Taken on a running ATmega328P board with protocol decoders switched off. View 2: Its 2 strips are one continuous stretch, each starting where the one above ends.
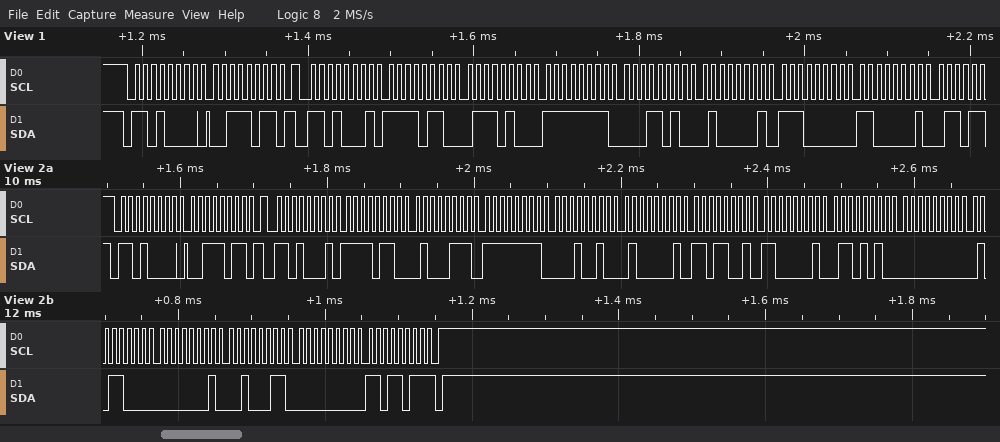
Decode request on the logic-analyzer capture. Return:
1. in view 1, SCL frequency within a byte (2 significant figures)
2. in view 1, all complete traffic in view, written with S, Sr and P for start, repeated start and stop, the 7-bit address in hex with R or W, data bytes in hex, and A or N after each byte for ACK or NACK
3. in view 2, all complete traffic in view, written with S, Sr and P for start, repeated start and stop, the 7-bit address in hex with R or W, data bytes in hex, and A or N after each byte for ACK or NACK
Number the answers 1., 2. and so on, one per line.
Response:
1. 100 kHz
2. S 68W A 3B A Sr 68R A F6 A 74 A FF A 1A A 41 A E0 A C1 A
3. S 68W A 3B A Sr 68R A F6 A 47 A FF A 12 A 41 A D9 A C1 A 6A A 00 A 58 A 01 A 23 A 00 A DB N P
